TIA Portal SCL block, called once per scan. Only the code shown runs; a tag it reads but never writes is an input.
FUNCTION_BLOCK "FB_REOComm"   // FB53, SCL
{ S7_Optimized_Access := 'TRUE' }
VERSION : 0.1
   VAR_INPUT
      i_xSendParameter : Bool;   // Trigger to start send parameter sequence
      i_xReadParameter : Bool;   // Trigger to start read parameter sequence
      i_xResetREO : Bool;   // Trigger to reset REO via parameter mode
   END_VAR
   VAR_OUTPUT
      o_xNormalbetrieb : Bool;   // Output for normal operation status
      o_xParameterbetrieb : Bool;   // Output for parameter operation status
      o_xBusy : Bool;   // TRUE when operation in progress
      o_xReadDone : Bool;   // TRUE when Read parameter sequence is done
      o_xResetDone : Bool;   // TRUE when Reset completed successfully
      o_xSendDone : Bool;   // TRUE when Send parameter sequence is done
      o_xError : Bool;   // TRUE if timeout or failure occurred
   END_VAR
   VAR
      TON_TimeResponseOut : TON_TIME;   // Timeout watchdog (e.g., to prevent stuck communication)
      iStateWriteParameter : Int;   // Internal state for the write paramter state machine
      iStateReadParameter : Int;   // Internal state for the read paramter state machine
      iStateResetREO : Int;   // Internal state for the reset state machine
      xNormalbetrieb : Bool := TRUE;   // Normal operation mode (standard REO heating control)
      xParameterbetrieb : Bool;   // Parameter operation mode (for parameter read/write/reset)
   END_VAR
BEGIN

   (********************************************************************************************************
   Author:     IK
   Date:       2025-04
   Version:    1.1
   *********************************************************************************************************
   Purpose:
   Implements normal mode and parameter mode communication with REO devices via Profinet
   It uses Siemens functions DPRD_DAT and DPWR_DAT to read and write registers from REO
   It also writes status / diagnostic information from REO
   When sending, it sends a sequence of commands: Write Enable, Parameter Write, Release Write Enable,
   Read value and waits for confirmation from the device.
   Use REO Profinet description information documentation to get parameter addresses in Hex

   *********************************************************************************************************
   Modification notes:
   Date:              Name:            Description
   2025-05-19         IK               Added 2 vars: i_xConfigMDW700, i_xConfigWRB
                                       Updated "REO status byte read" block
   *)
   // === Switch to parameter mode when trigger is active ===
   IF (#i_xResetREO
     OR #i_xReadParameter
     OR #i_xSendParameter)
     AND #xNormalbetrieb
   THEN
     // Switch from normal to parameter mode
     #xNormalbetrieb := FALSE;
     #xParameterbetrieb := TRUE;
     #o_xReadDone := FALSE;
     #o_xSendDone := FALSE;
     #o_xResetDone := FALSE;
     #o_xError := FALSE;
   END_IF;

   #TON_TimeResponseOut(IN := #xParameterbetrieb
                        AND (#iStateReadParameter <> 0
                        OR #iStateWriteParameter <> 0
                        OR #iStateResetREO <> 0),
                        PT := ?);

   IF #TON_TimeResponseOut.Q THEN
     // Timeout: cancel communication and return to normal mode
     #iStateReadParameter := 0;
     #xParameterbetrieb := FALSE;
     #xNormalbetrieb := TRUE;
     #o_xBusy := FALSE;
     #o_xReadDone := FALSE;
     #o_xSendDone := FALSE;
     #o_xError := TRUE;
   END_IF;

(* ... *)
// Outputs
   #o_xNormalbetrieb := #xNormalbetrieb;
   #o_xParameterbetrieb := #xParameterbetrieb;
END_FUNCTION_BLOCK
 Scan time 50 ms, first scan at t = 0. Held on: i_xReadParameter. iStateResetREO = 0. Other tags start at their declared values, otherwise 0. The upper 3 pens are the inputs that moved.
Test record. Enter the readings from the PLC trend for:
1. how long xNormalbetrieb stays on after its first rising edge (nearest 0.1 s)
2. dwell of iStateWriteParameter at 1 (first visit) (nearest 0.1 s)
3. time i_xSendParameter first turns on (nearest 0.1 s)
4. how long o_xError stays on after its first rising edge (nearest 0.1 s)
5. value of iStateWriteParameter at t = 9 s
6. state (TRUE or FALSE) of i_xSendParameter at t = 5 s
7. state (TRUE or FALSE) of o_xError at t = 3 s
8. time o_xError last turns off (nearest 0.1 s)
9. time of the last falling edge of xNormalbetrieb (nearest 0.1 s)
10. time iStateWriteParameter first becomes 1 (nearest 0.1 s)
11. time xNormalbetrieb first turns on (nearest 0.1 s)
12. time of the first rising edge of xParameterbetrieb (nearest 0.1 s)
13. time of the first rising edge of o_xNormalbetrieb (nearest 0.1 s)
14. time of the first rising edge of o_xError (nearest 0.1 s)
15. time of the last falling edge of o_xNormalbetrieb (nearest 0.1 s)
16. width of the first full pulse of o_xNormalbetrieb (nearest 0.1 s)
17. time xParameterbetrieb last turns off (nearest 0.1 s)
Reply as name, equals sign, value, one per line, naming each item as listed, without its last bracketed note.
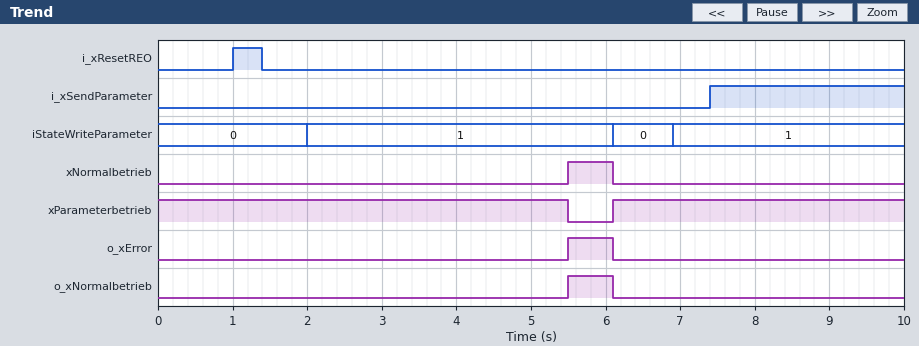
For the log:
how long xNormalbetrieb stays on after its first rising edge = 0.6 s
dwell of iStateWriteParameter at 1 (first visit) = 4.1 s
time i_xSendParameter first turns on = 7.4 s
how long o_xError stays on after its first rising edge = 0.6 s
value of iStateWriteParameter at t = 9 s = 1
state (TRUE or FALSE) of i_xSendParameter at t = 5 s = FALSE
state (TRUE or FALSE) of o_xError at t = 3 s = FALSE
time o_xError last turns off = 6.1 s
time of the last falling edge of xNormalbetrieb = 6.1 s
time iStateWriteParameter first becomes 1 = 2.0 s
time xNormalbetrieb first turns on = 5.5 s
time of the first rising edge of xParameterbetrieb = 6.1 s
time of the first rising edge of o_xNormalbetrieb = 5.5 s
time of the first rising edge of o_xError = 5.5 s
time of the last falling edge of o_xNormalbetrieb = 6.1 s
width of the first full pulse of o_xNormalbetrieb = 0.6 s
time xParameterbetrieb last turns off = 5.5 s
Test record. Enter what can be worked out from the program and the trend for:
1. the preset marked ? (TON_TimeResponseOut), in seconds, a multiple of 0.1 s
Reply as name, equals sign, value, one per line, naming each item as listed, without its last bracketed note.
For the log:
the preset marked ? (TON_TimeResponseOut), in seconds, a multiple of 0.1 s = 3.5 s
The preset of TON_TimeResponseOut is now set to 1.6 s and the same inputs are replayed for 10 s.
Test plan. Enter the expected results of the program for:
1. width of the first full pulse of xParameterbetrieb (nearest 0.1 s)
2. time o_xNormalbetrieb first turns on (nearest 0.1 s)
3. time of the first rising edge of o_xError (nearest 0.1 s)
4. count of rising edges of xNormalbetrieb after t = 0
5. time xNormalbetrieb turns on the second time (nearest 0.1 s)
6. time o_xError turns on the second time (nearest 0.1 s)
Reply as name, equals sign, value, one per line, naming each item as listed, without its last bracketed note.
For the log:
width of the first full pulse of xParameterbetrieb = 2.4 s
time o_xNormalbetrieb first turns on = 3.6 s
time of the first rising edge of o_xError = 3.6 s
count of rising edges of xNormalbetrieb after t = 0 = 2
time xNormalbetrieb turns on the second time = 8.5 s
time o_xError turns on the second time = 8.5 s
